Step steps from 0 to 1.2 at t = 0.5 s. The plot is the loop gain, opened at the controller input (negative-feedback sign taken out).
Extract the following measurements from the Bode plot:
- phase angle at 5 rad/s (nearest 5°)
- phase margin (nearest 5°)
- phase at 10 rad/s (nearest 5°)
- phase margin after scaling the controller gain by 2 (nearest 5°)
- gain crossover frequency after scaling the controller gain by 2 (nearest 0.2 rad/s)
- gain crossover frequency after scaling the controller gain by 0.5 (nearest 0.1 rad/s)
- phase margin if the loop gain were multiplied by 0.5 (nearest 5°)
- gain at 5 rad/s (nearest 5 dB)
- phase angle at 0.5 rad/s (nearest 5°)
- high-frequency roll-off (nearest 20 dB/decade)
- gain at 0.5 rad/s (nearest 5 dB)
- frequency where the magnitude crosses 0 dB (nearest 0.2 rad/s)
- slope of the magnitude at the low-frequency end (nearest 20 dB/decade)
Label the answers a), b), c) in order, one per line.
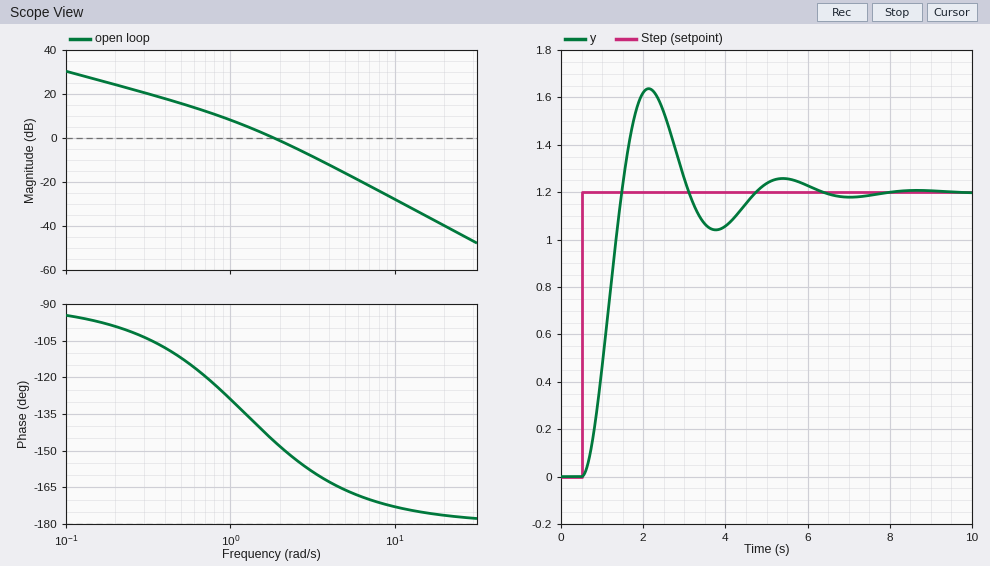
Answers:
a) -165°
b) 35°
c) -175°
d) 25°
e) 2.8 rad/s
f) 1.2 rad/s
g) 45°
h) -15 dB
i) -110°
j) -40 dB/decade
k) 15 dB
l) 1.8 rad/s
m) -20 dB/decade
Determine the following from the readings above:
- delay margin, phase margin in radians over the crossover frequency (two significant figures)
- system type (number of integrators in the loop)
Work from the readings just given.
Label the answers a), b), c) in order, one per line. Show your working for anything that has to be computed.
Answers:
a) 35 × π / 180 / 1.8 = 0.34 s
b) 1
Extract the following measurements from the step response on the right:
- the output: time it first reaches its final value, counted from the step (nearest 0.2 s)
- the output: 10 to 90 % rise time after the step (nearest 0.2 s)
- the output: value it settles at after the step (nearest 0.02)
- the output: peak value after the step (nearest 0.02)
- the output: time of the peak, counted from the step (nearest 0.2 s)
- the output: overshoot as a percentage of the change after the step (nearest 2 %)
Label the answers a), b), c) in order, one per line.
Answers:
a) 1.0 s
b) 0.6 s
c) 1.20
d) 1.64
e) 1.6 s
f) 36 %
